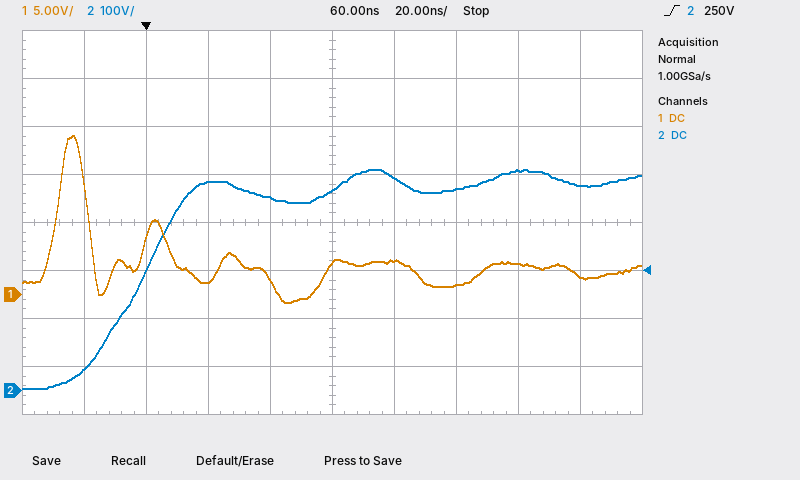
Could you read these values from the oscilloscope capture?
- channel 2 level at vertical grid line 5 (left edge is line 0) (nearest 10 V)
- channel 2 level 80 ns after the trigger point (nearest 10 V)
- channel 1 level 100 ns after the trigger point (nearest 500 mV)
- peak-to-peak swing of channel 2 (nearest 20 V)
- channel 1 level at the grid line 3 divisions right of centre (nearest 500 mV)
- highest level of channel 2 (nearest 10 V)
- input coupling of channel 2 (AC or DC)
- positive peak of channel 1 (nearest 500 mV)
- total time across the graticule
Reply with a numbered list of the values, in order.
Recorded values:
1. 420 V
2. 440 V
3. 1.0 V
4. 460 V
5. 3.0 V
6. 460 V
7. DC
8. 16.5 V
9. 200 ns
